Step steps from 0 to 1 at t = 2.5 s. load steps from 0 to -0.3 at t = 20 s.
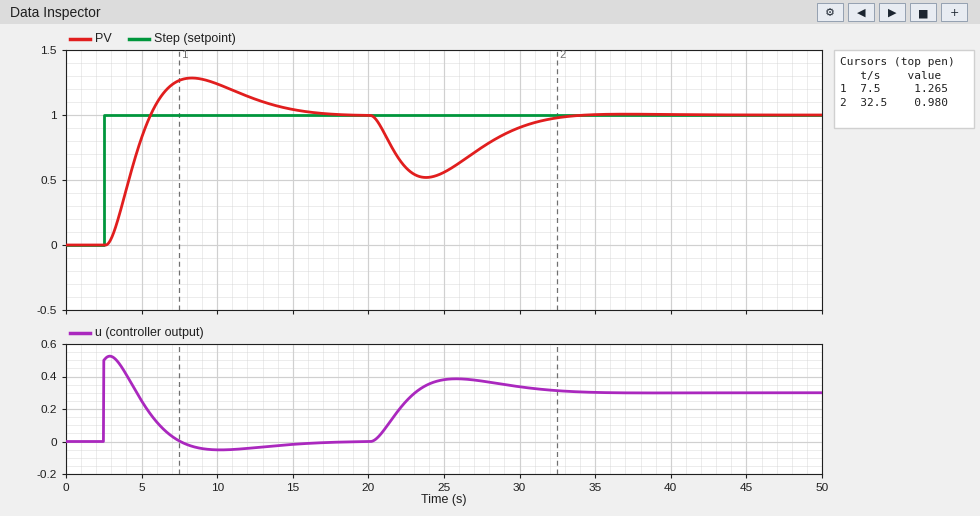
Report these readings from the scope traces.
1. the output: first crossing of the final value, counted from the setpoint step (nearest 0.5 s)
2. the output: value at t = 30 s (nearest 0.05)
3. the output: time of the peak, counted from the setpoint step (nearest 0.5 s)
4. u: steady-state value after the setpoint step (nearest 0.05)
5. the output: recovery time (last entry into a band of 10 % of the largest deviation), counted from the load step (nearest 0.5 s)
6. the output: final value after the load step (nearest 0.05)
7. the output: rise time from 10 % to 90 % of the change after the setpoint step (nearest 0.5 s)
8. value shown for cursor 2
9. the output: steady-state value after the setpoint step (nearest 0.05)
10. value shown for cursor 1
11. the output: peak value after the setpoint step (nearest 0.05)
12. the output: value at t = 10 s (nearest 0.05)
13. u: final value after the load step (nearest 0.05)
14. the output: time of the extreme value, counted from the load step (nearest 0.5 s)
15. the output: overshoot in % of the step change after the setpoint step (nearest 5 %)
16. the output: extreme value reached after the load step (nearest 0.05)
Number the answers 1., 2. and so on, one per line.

1. 3.0 s
2. 0.90
3. 6.0 s
4. 0.00
5. 11.5 s
6. 1.00
7. 2.0 s
8. 0.980
9. 1.00
10. 1.265
11. 1.30
12. 1.25
13. 0.30
14. 4.0 s
15. 30 %
16. 0.50
